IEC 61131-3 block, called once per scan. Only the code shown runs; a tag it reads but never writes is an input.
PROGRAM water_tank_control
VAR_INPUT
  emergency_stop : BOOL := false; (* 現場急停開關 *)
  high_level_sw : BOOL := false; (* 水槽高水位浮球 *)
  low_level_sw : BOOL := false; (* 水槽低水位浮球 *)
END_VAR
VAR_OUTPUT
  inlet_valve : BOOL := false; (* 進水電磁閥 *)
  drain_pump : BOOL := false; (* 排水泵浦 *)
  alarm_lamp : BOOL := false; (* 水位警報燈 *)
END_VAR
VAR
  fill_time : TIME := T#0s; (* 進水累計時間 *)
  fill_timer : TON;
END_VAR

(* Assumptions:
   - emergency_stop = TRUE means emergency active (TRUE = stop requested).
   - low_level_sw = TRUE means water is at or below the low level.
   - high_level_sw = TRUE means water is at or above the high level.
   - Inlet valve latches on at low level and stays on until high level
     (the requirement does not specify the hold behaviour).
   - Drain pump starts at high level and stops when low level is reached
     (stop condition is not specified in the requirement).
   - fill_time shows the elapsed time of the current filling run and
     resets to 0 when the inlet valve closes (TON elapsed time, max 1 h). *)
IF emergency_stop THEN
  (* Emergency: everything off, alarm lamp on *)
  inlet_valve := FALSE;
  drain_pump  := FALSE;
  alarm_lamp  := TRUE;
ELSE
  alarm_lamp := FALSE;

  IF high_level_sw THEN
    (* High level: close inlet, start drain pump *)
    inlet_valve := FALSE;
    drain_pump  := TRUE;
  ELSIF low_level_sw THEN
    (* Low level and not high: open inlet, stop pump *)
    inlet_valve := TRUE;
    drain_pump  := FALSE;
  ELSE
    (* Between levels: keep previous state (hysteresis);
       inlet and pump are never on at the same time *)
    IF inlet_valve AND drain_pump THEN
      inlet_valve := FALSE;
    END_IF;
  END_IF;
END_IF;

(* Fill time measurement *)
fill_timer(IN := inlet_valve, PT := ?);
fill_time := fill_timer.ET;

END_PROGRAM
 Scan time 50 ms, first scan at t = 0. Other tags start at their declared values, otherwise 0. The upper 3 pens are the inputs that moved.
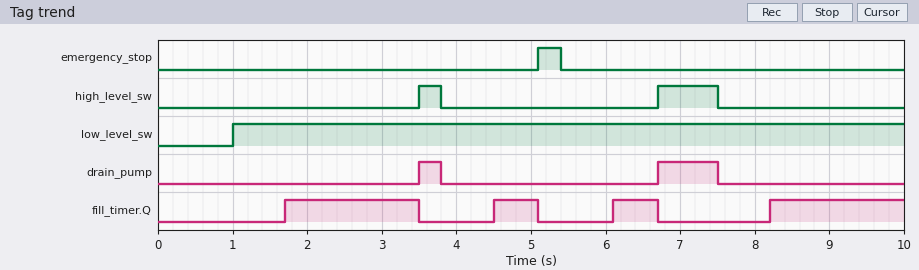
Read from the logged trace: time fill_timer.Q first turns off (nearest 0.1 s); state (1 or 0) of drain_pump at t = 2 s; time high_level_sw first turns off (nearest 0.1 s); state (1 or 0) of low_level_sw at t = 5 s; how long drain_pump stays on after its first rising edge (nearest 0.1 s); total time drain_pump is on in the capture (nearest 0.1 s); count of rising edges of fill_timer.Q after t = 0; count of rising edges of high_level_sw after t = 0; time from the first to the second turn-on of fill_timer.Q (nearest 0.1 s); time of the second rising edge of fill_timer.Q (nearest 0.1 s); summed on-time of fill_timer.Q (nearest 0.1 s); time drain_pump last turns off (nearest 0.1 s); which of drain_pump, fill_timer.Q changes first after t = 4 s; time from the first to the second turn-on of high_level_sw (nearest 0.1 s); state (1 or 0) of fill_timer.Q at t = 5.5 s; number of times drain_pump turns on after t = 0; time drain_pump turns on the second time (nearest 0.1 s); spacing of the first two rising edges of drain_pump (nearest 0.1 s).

3.5 s
0
3.8 s
1
0.3 s
1.1 s
4
2
2.8 s
4.5 s
4.8 s
7.5 s
fill_timer.Q
3.2 s
0
2
6.7 s
3.2 s
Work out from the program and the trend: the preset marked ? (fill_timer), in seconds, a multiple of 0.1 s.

0.7 s
